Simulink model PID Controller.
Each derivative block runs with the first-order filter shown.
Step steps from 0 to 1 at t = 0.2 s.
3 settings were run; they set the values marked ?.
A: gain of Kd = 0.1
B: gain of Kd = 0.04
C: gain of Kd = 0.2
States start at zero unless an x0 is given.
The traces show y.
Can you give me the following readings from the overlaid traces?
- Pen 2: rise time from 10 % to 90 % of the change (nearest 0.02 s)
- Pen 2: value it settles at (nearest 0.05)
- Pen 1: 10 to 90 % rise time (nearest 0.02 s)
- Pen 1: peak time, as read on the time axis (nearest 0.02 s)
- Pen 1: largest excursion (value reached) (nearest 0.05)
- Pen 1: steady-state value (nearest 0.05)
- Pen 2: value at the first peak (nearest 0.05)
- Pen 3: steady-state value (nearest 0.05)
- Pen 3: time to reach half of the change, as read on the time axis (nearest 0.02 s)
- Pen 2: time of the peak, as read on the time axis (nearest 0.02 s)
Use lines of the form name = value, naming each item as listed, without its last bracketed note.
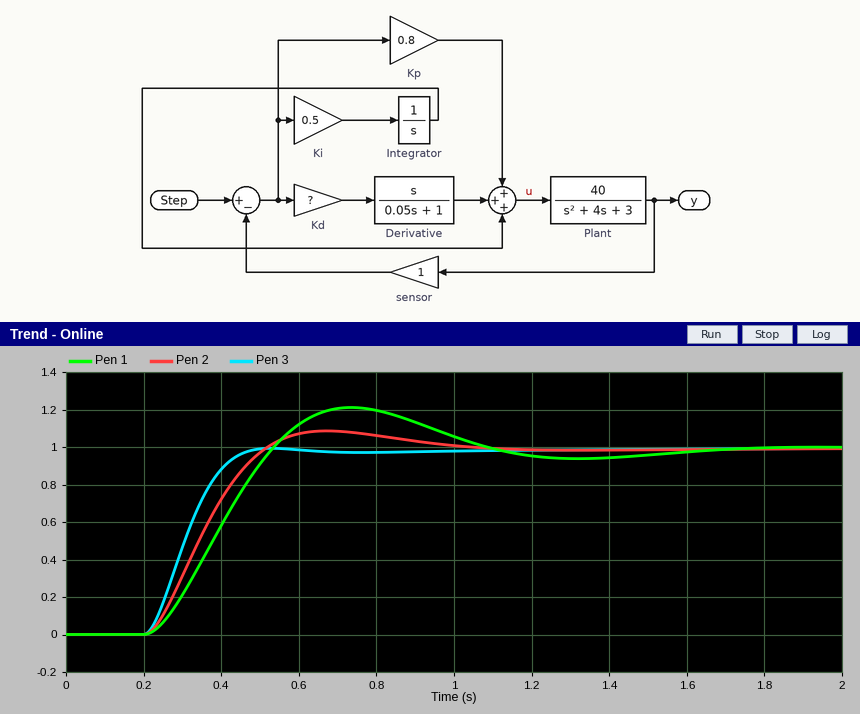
Pen 2: rise time from 10 % to 90 % of the change = 0.22 s
Pen 2: value it settles at = 1.00
Pen 1: 10 to 90 % rise time = 0.24 s
Pen 1: peak time, as read on the time axis = 0.74 s
Pen 1: largest excursion (value reached) = 1.20
Pen 1: steady-state value = 1.00
Pen 2: value at the first peak = 1.10
Pen 3: steady-state value = 1.00
Pen 3: time to reach half of the change, as read on the time axis = 0.30 s
Pen 2: time of the peak, as read on the time axis = 0.68 s
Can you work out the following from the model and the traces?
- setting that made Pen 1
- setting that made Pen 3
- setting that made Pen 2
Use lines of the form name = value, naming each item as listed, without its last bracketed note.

setting that made Pen 1 = B
setting that made Pen 3 = C
setting that made Pen 2 = A
